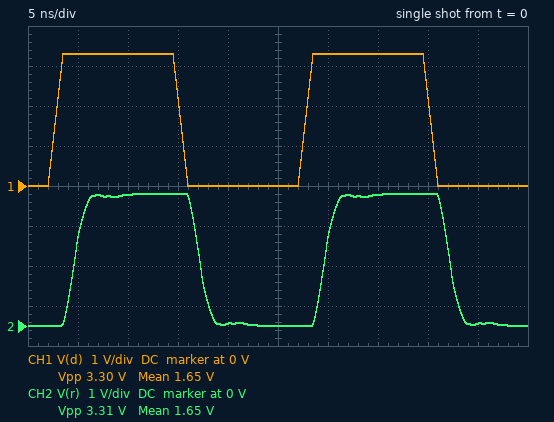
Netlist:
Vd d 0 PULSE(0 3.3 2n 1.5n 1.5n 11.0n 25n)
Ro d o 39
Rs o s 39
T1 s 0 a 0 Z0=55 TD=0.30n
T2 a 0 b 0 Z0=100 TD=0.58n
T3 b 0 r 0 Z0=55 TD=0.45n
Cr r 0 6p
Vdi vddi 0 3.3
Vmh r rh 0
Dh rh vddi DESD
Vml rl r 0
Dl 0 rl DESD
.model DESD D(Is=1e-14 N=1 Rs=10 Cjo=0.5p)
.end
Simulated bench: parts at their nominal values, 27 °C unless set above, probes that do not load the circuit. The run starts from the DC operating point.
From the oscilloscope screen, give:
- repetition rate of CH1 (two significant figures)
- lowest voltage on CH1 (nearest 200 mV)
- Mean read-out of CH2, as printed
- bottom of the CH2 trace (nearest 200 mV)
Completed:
40 MHz
0 V
1.65 V
0 V
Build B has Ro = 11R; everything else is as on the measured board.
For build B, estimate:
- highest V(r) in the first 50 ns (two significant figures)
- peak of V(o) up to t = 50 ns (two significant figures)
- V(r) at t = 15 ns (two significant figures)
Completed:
4.0 V
3.4 V
3.3 V
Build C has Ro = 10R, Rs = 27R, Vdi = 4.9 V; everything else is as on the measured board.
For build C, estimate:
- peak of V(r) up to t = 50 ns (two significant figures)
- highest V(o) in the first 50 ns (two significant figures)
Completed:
4.6 V
3.4 V
